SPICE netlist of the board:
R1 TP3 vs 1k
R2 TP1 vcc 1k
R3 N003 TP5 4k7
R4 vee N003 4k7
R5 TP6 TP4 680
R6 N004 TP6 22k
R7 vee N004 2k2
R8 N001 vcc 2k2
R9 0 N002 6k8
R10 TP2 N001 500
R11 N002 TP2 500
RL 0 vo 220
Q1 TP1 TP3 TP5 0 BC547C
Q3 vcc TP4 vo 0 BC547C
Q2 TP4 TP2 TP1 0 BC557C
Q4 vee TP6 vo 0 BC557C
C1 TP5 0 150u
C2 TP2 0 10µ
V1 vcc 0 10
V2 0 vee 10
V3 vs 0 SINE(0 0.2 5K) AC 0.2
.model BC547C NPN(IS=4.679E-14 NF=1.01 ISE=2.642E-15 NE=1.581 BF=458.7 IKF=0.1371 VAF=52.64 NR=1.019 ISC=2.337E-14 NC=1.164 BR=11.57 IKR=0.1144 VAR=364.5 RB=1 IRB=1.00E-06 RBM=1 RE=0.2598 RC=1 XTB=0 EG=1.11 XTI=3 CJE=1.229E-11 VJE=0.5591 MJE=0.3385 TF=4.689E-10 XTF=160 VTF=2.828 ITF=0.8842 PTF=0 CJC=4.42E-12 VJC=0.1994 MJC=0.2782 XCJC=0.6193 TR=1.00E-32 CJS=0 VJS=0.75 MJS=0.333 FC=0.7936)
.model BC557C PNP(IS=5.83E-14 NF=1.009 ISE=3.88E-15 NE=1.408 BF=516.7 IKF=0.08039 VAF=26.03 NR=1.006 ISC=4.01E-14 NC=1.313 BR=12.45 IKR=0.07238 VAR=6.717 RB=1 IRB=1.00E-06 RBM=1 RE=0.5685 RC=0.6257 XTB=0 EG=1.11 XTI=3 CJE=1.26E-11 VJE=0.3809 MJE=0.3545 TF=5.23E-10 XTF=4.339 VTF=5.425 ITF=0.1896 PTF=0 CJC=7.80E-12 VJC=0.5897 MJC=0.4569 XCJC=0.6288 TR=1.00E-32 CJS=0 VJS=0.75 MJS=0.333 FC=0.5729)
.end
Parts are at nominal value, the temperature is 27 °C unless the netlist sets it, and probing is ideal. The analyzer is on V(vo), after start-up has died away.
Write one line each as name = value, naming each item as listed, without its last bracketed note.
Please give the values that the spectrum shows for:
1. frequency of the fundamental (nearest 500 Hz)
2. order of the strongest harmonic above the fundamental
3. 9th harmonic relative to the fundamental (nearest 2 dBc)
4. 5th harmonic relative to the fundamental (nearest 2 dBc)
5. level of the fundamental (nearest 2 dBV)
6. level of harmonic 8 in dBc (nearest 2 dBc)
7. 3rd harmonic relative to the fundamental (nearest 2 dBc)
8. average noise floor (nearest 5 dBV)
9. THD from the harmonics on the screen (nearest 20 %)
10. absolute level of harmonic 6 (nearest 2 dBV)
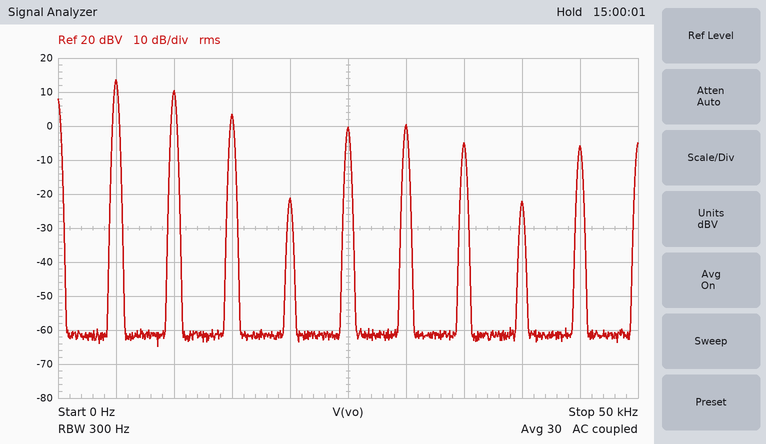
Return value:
frequency of the fundamental = 5.0 kHz
order of the strongest harmonic above the fundamental = 2
9th harmonic relative to the fundamental = -20 dBc
5th harmonic relative to the fundamental = -14 dBc
level of the fundamental = 14 dBV
level of harmonic 8 in dBc = -36 dBc
3rd harmonic relative to the fundamental = -10 dBc
average noise floor = -60 dBV
THD from the harmonics on the screen = 80 %
absolute level of harmonic 6 = 0 dBV
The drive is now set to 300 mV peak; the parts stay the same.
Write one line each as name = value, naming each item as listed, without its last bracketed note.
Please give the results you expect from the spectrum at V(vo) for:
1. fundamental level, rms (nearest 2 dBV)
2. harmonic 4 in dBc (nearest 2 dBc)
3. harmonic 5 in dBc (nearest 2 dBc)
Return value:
fundamental level, rms = 12 dBV
harmonic 4 in dBc = -18 dBc
harmonic 5 in dBc = -20 dBc
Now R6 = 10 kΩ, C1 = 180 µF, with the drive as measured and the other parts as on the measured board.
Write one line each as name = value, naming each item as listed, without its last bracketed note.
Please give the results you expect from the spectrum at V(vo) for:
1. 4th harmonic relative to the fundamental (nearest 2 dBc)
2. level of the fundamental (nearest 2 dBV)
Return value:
4th harmonic relative to the fundamental = -32 dBc
level of the fundamental = 14 dBV
